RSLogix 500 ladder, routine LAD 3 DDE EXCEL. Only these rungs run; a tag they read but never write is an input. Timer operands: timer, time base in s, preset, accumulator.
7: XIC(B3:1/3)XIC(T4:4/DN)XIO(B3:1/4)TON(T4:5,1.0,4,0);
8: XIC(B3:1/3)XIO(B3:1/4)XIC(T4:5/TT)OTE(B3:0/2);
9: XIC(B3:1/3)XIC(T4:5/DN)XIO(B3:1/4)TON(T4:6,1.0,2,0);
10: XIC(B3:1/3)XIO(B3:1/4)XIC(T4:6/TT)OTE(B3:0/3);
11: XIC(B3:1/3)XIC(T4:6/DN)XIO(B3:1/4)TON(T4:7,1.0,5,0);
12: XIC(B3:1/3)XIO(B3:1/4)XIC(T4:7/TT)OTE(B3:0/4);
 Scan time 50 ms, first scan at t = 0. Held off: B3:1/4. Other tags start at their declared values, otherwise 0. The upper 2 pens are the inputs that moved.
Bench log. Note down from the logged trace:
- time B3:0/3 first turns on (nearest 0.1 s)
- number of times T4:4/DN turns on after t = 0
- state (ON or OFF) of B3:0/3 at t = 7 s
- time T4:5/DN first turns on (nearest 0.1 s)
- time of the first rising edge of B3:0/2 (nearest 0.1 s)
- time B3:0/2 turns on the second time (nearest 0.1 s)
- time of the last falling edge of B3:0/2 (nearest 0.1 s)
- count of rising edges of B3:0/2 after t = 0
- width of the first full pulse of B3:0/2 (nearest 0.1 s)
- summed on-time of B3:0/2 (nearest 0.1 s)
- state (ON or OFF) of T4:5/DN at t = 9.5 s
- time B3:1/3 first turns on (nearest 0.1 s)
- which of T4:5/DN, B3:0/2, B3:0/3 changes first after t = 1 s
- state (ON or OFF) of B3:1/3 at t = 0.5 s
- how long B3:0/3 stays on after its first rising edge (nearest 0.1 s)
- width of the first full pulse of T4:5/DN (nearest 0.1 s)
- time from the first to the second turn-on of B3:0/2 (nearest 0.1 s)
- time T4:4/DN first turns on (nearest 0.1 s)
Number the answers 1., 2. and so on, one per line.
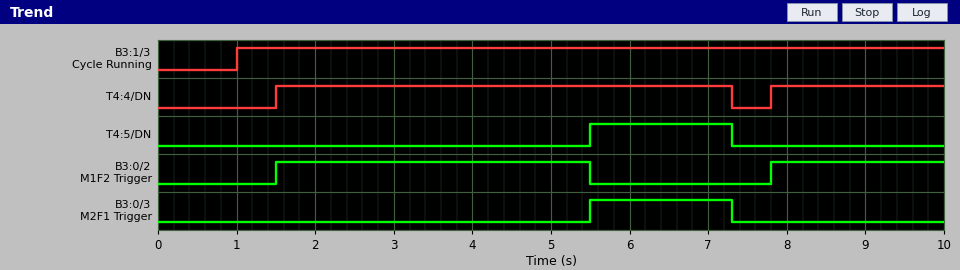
1. 5.5 s
2. 2
3. ON
4. 5.5 s
5. 1.5 s
6. 7.8 s
7. 5.5 s
8. 2
9. 4.0 s
10. 6.2 s
11. OFF
12. 1.0 s
13. B3:0/2
14. OFF
15. 1.8 s
16. 1.8 s
17. 6.3 s
18. 1.5 s
